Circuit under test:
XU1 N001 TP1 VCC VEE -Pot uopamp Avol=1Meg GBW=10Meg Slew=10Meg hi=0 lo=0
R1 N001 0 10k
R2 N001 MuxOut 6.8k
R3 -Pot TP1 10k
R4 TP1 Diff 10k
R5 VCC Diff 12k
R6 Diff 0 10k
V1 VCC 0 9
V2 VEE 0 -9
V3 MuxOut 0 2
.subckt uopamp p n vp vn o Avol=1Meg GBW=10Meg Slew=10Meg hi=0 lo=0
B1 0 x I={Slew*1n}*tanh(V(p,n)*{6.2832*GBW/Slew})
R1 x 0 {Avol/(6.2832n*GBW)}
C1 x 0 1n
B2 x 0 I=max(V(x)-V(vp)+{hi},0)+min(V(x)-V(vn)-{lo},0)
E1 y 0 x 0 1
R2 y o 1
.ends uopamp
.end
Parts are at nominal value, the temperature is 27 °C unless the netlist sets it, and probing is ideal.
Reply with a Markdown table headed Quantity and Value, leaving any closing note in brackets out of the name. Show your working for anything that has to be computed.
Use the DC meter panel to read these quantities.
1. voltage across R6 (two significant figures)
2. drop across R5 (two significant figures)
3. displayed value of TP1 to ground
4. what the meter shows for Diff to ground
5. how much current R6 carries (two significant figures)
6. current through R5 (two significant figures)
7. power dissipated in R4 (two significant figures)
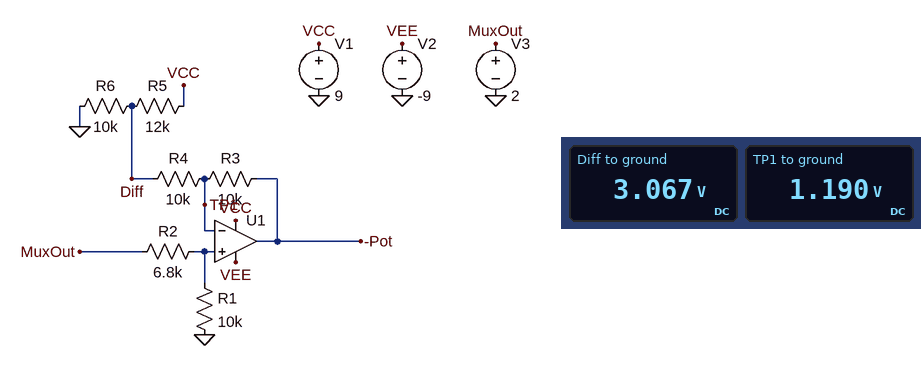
| Quantity | Value |
|---|---|
| voltage across R6 | 3.067 V = 3.1 V |
| drop across R5 | 9 V - 3.067 V = 5.9 V |
| displayed value of TP1 to ground | 1.190 V |
| what the meter shows for Diff to ground | 3.067 V |
| how much current R6 carries | (3.067 V) / 10 kΩ = 310 µA |
| current through R5 | (9 V - 3.067 V) / 12 kΩ = 490 µA |
| power dissipated in R4 | (3.067 V - 1.19 V)^2 / 10 kΩ = 350 µW |
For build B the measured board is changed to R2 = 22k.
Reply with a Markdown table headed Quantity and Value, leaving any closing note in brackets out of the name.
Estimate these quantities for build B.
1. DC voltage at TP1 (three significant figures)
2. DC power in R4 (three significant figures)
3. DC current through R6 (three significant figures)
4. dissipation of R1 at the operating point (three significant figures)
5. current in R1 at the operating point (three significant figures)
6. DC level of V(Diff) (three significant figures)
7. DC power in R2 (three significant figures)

| Quantity | Value |
|---|---|
| DC voltage at TP1 | 625 mV |
| DC power in R4 | 503 µW |
| DC current through R6 | 287 µA |
| dissipation of R1 at the operating point | 39.1 µW |
| current in R1 at the operating point | 62.5 µA |
| DC level of V(Diff) | 2.87 V |
| DC power in R2 | 85.9 µW |
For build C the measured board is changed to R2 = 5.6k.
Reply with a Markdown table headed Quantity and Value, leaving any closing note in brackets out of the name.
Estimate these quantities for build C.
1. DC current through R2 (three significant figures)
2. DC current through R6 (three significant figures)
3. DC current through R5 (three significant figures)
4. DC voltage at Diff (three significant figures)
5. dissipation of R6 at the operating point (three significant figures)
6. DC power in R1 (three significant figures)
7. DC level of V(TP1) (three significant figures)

| Quantity | Value |
|---|---|
| DC current through R2 | 128 µA |
| DC current through R6 | 310 µA |
| DC current through R5 | 492 µA |
| DC voltage at Diff | 3.10 V |
| dissipation of R6 at the operating point | 961 µW |
| DC power in R1 | 164 µW |
| DC level of V(TP1) | 1.28 V |
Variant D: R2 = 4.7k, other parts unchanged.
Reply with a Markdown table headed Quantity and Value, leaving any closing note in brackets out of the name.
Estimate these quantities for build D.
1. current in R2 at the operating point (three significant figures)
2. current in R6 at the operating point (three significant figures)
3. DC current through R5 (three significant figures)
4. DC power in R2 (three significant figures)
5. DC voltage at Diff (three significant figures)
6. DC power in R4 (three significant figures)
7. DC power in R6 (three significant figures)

| Quantity | Value |
|---|---|
| current in R2 at the operating point | 136 µA |
| current in R6 at the operating point | 313 µA |
| DC current through R5 | 489 µA |
| DC power in R2 | 87.0 µW |
| DC voltage at Diff | 3.13 V |
| DC power in R4 | 312 µW |
| DC power in R6 | 978 µW |
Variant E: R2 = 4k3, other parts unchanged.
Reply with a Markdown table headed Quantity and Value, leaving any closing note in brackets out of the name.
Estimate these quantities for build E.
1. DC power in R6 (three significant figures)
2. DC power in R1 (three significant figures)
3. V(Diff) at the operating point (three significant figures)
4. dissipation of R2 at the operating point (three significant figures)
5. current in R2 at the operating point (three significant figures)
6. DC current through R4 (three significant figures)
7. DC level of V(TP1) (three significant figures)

| Quantity | Value |
|---|---|
| DC power in R6 | 986 µW |
| DC power in R1 | 196 µW |
| V(Diff) at the operating point | 3.14 V |
| dissipation of R2 at the operating point | 84.1 µW |
| current in R2 at the operating point | 140 µA |
| DC current through R4 | 174 µA |
| DC level of V(TP1) | 1.40 V |
